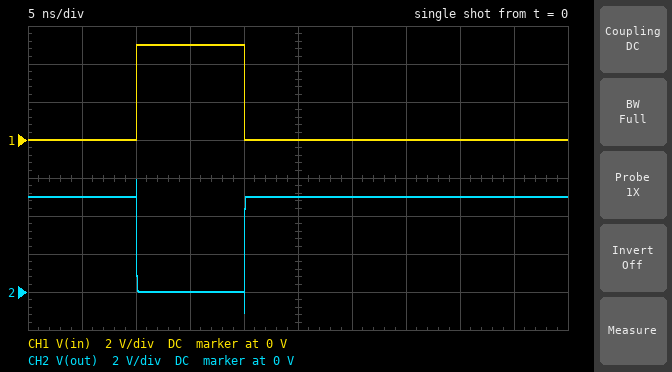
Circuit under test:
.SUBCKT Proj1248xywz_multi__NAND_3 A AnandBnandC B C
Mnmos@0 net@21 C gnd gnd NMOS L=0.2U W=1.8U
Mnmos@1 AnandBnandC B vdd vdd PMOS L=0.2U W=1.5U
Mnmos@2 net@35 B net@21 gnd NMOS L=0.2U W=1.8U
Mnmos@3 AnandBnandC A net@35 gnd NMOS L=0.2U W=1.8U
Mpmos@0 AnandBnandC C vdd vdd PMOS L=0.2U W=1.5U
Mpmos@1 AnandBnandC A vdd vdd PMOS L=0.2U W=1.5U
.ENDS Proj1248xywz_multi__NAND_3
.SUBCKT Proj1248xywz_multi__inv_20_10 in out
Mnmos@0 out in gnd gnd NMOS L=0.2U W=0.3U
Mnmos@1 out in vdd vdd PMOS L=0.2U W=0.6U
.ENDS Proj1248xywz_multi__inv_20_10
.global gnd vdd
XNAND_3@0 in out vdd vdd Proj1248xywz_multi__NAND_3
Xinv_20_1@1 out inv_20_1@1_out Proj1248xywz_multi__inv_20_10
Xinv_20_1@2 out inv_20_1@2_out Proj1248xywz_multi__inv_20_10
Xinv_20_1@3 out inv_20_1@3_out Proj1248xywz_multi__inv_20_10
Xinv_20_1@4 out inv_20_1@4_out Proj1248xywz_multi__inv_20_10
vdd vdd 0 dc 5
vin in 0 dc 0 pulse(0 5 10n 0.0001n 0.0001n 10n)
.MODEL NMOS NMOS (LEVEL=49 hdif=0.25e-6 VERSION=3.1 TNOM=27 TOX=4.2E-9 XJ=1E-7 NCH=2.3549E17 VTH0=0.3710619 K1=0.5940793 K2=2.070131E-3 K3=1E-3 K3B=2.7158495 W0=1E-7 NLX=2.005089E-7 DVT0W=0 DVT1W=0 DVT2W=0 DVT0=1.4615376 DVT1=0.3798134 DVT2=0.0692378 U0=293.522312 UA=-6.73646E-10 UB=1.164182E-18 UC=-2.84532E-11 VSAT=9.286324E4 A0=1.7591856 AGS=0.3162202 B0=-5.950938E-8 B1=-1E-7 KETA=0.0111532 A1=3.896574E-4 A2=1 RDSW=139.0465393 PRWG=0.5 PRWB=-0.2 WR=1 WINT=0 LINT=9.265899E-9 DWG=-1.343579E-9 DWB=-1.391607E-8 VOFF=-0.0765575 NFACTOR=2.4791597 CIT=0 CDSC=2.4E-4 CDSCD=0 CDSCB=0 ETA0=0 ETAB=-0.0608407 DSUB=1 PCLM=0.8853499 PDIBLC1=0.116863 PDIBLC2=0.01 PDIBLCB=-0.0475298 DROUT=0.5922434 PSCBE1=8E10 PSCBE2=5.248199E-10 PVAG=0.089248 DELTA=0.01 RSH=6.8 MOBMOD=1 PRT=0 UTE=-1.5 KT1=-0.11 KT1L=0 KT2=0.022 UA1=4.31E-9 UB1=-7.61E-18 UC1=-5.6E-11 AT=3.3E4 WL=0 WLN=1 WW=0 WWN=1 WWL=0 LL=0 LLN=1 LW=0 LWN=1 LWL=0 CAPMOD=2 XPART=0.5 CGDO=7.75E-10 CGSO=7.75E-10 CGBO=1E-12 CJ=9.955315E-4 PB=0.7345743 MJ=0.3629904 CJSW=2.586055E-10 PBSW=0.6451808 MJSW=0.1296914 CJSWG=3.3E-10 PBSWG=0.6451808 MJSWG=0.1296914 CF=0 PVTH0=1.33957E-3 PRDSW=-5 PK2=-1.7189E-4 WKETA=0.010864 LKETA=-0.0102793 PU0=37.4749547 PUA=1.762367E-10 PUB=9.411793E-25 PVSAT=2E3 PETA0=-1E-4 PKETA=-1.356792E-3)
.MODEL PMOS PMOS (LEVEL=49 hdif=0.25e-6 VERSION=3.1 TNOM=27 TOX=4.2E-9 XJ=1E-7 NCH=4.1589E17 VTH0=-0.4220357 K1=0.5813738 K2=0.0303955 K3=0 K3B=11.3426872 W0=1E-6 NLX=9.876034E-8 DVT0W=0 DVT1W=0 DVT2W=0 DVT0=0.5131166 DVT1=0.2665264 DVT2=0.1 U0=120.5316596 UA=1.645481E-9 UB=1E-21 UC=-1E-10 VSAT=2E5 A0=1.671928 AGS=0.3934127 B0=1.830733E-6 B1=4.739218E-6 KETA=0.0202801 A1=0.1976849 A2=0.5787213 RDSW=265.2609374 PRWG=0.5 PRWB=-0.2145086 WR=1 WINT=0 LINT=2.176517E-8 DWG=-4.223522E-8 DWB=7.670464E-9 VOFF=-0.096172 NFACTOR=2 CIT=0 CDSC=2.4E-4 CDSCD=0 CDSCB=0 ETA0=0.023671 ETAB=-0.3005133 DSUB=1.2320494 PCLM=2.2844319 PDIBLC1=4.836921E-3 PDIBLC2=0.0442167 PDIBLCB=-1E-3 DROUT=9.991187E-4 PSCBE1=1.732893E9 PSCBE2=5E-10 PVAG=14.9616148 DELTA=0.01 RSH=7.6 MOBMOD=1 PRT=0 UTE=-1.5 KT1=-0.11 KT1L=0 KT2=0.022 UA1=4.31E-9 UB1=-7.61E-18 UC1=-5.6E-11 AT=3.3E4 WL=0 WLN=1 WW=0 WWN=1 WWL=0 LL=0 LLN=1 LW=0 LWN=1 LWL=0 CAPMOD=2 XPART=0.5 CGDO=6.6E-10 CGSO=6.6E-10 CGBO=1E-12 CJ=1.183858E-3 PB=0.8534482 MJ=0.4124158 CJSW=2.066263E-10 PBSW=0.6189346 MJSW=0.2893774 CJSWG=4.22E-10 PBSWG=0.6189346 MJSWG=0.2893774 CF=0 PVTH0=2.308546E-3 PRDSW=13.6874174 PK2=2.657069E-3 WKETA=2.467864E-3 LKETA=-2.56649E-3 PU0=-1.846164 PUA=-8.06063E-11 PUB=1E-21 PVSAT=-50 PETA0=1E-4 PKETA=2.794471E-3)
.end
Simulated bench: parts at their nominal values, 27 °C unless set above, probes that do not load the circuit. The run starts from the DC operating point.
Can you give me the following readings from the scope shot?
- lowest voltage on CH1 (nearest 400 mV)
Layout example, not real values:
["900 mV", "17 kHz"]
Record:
["0 V"]
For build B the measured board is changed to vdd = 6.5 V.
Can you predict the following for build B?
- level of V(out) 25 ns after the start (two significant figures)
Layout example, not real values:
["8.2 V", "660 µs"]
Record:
["6.5 V"]
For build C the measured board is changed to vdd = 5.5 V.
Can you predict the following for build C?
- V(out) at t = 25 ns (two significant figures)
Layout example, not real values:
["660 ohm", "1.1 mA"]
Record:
["5.5 V"]
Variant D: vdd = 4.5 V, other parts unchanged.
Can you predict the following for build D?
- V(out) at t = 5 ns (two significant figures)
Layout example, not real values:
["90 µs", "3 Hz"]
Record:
["4.5 V"]
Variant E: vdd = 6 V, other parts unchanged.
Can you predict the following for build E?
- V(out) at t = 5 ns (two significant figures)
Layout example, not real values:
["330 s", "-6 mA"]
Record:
["6.0 V"]
